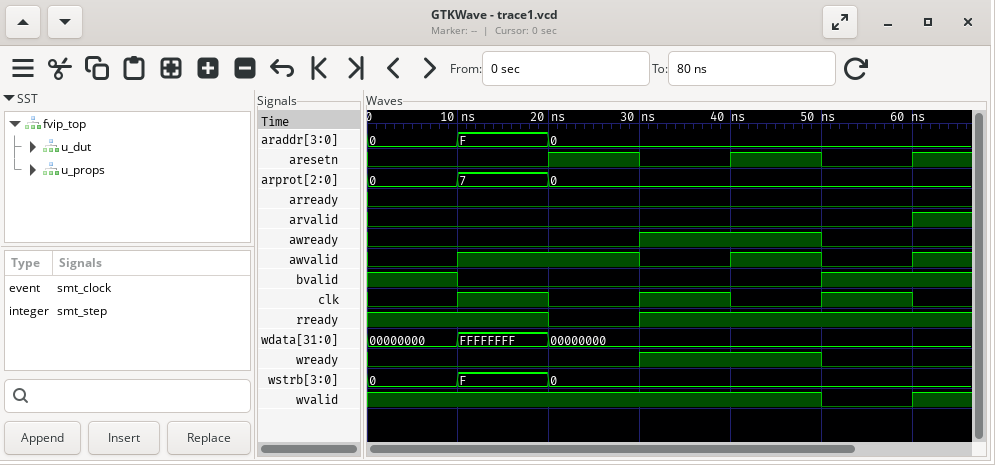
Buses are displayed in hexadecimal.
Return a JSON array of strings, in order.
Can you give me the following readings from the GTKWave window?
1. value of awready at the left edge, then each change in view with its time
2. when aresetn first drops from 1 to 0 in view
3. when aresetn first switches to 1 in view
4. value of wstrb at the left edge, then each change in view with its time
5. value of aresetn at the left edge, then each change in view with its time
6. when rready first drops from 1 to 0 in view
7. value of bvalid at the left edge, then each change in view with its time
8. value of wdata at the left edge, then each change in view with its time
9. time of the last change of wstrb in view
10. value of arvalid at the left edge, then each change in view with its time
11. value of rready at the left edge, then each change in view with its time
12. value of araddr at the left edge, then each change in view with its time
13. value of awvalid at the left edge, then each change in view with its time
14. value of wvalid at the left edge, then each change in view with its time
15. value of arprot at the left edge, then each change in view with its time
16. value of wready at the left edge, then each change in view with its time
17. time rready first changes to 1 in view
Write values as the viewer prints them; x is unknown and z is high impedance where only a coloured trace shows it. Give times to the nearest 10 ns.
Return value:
["0, 1 at 30 ns, 0 at 50 ns", "30 ns", "20 ns", "0, F at 10 ns, 0 at 20 ns", "0, 1 at 20 ns, 0 at 30 ns, 1 at 40 ns, 0 at 50 ns, 1 at 60 ns", "20 ns", "1, 0 at 10 ns, 1 at 50 ns", "00000000, FFFFFFFF at 10 ns, 00000000 at 20 ns", "20 ns", "0, 1 at 60 ns", "1, 0 at 20 ns, 1 at 30 ns", "0, F at 10 ns, 0 at 20 ns", "0, 1 at 10 ns, 0 at 30 ns, 1 at 40 ns, 0 at 50 ns, 1 at 60 ns", "1, 0 at 50 ns, 1 at 60 ns", "0, 7 at 10 ns, 0 at 20 ns", "0, 1 at 30 ns, 0 at 50 ns", "30 ns"]
